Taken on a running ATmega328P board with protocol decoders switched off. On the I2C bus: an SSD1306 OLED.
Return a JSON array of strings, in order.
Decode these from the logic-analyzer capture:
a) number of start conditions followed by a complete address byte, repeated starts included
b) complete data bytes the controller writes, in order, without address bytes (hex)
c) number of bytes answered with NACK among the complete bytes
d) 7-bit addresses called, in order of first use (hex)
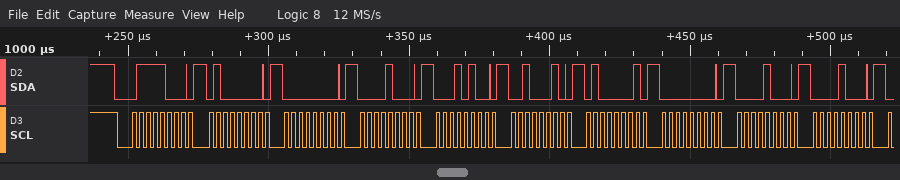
["1", "40 00 08 14 22 41 00 08 08", "0", "0x3C"]
